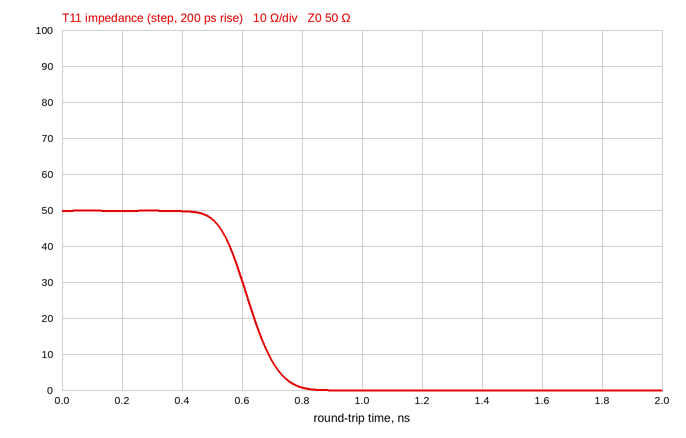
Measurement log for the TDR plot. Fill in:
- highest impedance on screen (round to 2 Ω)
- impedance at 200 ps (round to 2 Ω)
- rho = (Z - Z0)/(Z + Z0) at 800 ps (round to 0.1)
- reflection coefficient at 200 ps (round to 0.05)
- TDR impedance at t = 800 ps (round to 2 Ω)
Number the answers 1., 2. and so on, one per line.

1. 50 Ω
2. 50 Ω
3. -1.0
4. 0.00
5. 0 Ω
